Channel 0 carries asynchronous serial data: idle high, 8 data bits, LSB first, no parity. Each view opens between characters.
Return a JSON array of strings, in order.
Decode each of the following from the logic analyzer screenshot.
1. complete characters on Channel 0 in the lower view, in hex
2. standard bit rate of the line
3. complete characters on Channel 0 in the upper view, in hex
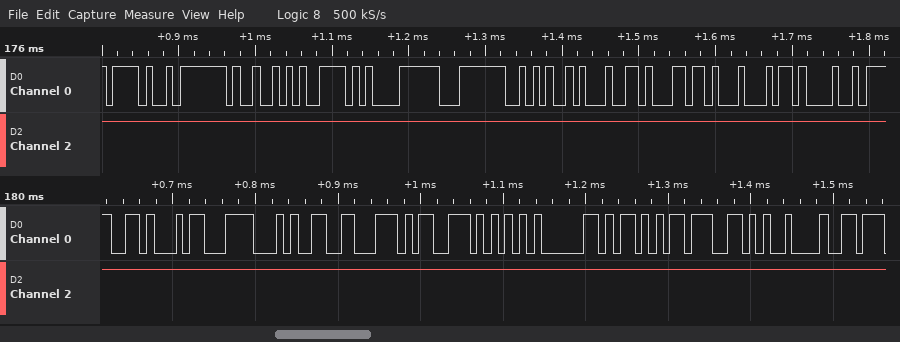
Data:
["16, E3, 94, C6, CD, 55, 60, AB, 67, 09", "115200 baud", "2F, 7F, 52, 5E, F8, FC, 2A, 91, B1, 11, 0B"]
